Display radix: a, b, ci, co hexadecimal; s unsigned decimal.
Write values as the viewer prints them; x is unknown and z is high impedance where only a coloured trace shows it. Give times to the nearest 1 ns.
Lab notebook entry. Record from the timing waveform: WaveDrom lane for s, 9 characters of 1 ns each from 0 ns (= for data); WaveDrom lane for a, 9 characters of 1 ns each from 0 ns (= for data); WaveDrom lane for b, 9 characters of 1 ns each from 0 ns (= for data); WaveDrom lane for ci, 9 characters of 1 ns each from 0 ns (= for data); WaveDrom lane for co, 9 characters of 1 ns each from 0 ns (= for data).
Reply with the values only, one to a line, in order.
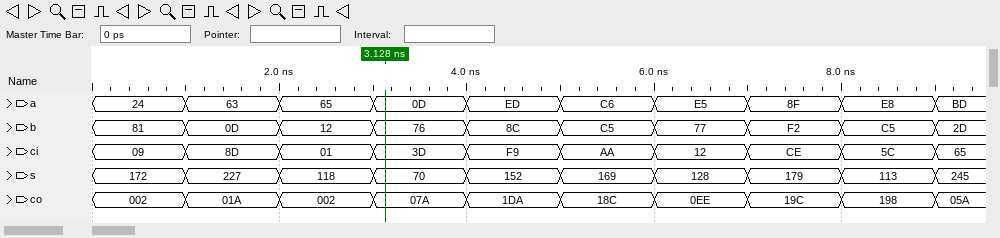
{name: 's', wave: '=========', data: '172 227 118 70 152 169 128 179 113'}
{name: 'a', wave: '=========', data: '24 63 65 0D ED C6 E5 8F E8'}
{name: 'b', wave: '=========', data: '81 0D 12 76 8C C5 77 F2 C5'}
{name: 'ci', wave: '=========', data: '09 8D 01 3D F9 AA 12 CE 5C'}
{name: 'co', wave: '=========', data: '002 01A 002 07A 1DA 18C 0EE 19C 198'}
